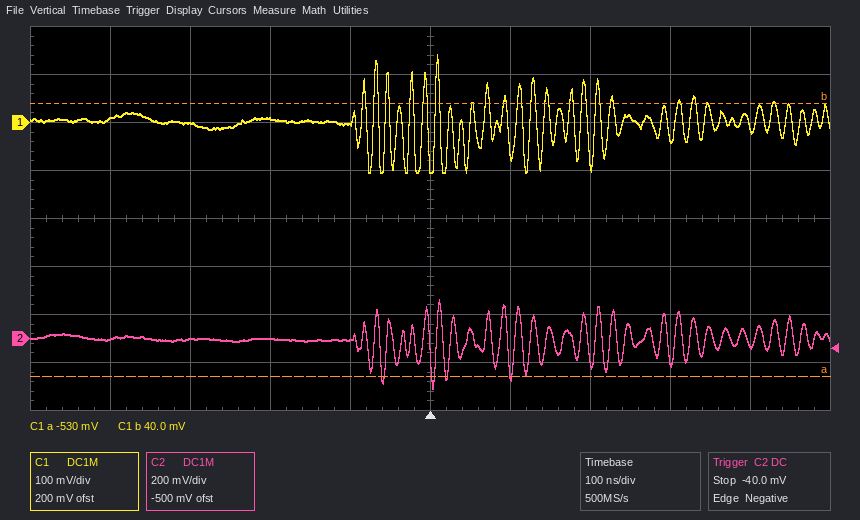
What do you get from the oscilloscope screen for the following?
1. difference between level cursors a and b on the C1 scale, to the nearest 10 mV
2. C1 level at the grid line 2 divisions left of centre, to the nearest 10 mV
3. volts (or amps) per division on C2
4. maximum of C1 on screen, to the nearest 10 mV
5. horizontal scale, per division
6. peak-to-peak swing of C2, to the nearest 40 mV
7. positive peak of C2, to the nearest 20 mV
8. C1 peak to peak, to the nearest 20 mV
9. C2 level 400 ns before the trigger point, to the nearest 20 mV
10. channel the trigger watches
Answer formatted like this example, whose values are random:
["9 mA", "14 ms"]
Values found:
["570 mV", "10 mV", "200 mV", "140 mV", "100 ns", "360 mV", "160 mV", "240 mV", "0 mV", "C2"]
